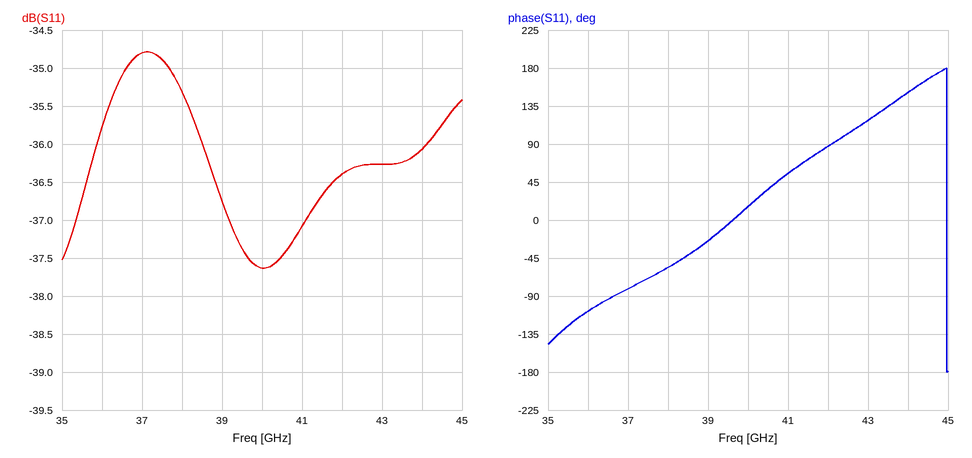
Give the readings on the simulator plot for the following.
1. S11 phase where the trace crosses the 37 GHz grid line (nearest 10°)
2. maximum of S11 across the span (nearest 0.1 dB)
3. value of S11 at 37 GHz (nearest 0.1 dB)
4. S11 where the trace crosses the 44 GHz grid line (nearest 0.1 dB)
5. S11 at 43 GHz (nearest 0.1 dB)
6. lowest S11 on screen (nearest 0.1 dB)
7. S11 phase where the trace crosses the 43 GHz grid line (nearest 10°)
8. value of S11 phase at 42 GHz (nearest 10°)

-80°
-34.8 dB
-34.8 dB
-36.1 dB
-36.3 dB
-37.6 dB
120°
90°
